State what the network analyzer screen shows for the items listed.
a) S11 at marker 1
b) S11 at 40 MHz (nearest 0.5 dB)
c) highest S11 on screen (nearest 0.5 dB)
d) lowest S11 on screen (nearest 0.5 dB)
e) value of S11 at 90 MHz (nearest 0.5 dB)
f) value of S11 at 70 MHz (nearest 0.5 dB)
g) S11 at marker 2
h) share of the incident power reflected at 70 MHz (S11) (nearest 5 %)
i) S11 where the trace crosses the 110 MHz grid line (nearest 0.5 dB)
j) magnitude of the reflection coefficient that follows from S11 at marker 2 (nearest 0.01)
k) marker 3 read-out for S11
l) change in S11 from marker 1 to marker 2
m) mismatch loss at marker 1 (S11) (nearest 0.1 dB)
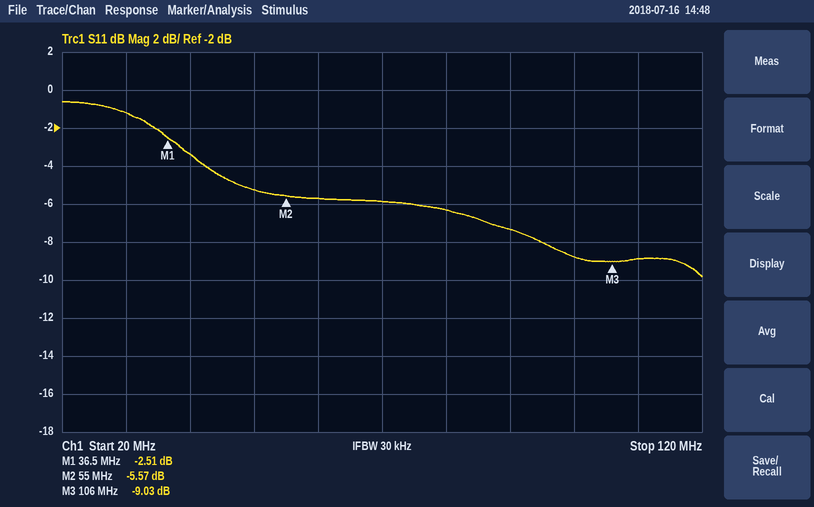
-2.51 dB
-3.5 dB
-0.5 dB
-10.0 dB
-7.5 dB
-6.0 dB
-5.57 dB
25 %
-9.0 dB
0.53
-9.03 dB
-3.06 dB
3.6 dB
